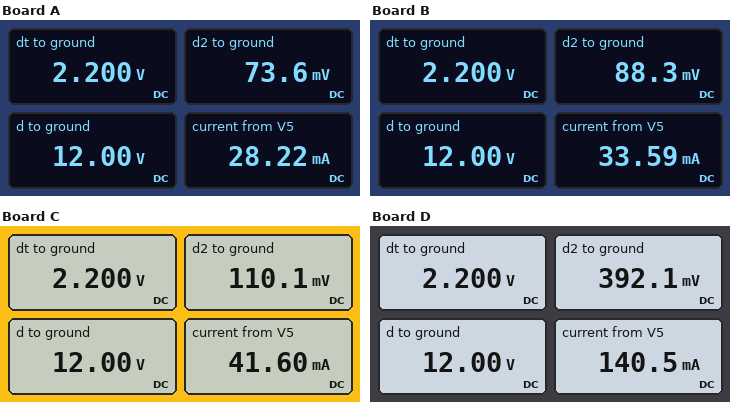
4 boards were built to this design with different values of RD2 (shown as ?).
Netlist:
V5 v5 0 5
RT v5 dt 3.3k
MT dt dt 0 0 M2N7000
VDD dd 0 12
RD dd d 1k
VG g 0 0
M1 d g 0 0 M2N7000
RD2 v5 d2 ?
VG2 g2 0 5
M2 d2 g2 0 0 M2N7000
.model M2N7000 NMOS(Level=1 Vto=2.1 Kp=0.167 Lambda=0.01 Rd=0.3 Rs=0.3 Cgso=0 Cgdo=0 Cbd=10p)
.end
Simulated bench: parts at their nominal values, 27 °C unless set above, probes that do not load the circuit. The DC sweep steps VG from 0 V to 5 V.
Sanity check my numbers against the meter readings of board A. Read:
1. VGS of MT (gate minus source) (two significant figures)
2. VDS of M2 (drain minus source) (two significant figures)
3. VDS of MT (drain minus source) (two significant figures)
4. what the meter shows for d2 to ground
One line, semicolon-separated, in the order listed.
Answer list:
2.2 V; 74 mV; 2.2 V; 73.6 mV
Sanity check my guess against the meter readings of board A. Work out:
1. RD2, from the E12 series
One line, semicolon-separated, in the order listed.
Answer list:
180 Ω
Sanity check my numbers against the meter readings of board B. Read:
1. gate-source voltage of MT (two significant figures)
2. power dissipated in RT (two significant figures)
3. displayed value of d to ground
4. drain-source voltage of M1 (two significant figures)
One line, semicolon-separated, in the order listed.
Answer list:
2.2 V; 2.4 mW; 12.00 V; 12 V
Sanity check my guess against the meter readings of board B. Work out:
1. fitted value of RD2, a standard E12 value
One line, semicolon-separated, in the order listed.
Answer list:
150 Ω
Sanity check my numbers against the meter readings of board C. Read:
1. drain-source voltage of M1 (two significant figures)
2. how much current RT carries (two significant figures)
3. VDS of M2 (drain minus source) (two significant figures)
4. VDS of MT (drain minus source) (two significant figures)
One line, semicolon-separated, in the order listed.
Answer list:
12 V; 850 µA; 110 mV; 2.2 V
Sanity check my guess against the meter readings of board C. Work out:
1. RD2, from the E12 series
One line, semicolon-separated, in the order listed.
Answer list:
120 Ω
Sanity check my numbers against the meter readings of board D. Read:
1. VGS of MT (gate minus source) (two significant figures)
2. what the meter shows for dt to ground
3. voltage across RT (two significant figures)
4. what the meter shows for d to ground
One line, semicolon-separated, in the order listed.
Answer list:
2.2 V; 2.200 V; 2.8 V; 12.00 V
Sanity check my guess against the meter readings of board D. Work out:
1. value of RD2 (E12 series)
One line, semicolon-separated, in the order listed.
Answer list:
33 Ω
